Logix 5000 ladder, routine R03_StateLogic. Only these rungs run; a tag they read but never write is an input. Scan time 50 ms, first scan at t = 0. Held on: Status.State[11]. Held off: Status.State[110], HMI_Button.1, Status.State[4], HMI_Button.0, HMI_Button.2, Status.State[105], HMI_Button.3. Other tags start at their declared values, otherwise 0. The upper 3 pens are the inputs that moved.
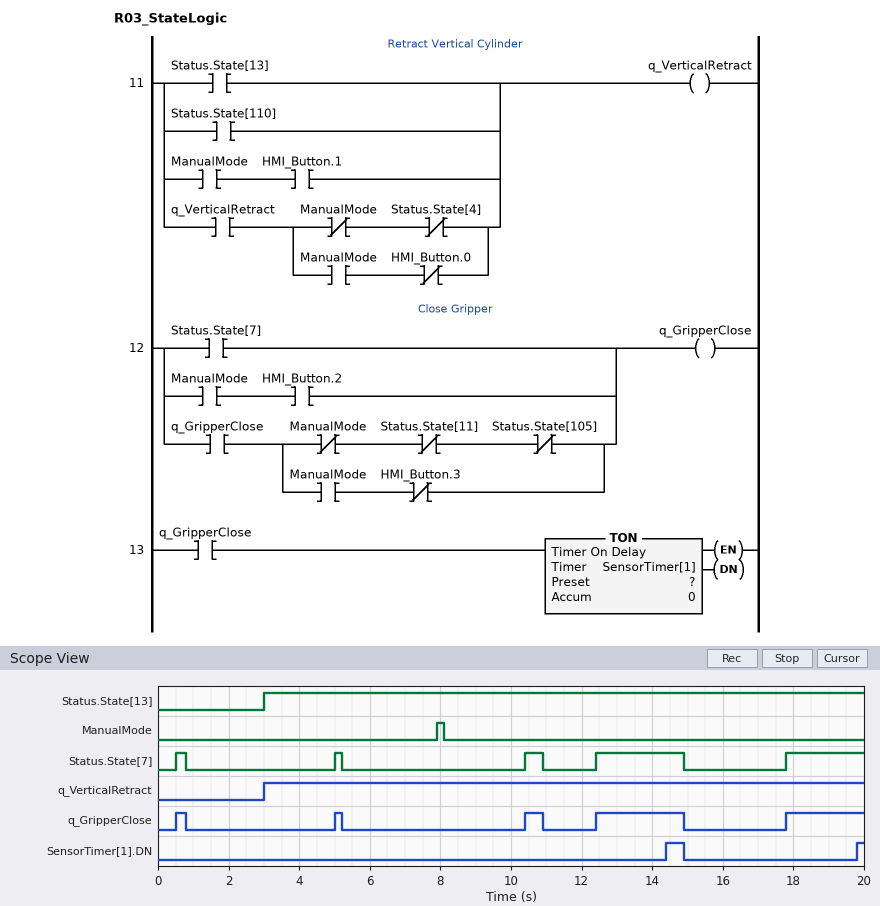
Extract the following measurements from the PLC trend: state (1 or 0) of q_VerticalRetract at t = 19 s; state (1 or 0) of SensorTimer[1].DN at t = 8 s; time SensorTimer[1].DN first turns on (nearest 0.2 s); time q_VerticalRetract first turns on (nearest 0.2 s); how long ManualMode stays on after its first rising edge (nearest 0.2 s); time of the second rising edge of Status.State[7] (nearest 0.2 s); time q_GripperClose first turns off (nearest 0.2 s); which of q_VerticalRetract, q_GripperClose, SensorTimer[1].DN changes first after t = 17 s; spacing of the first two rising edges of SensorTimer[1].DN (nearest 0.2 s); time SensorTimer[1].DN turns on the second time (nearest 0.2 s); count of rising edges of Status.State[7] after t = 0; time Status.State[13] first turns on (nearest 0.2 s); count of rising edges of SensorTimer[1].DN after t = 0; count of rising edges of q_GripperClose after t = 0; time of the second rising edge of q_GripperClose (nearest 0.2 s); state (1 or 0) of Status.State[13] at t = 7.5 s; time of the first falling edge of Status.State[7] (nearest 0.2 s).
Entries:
1
0
14.4 s
3.0 s
0.2 s
5.0 s
0.8 s
q_GripperClose
5.4 s
19.8 s
5
3.0 s
2
5
5.0 s
1
0.8 s
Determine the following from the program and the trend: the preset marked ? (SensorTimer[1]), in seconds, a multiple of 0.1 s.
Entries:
2.0 s
